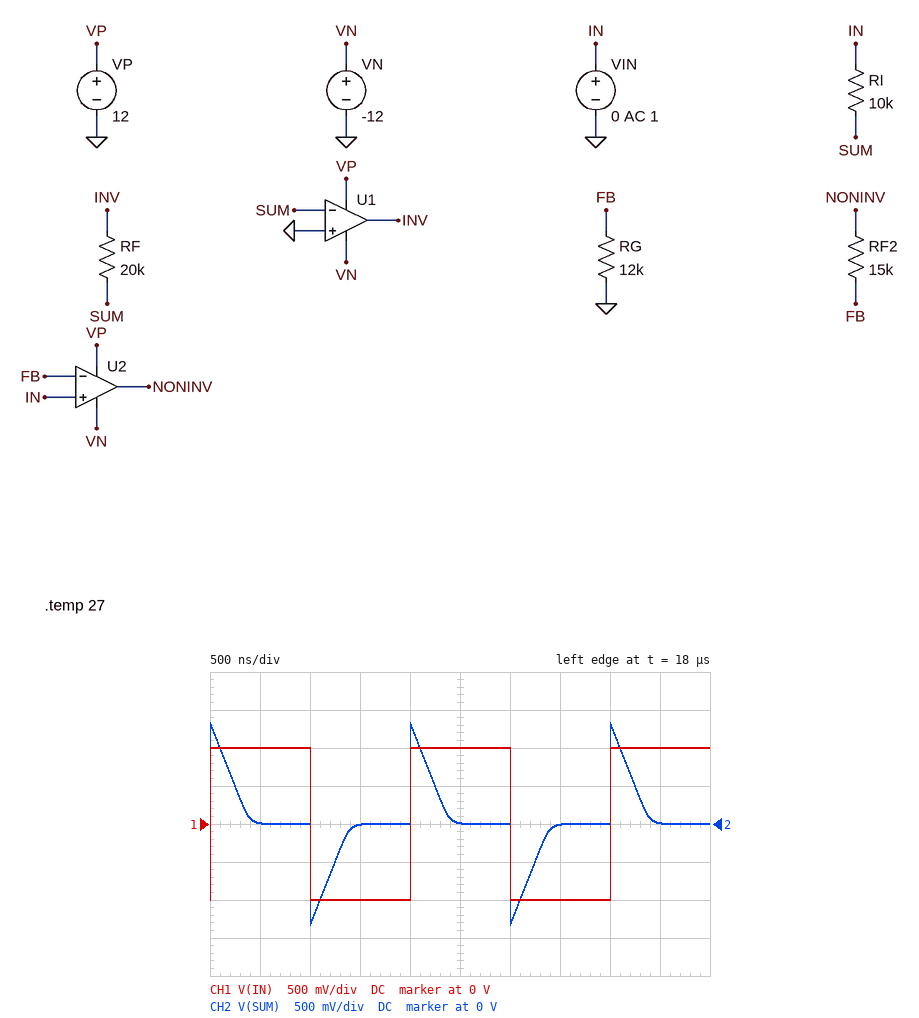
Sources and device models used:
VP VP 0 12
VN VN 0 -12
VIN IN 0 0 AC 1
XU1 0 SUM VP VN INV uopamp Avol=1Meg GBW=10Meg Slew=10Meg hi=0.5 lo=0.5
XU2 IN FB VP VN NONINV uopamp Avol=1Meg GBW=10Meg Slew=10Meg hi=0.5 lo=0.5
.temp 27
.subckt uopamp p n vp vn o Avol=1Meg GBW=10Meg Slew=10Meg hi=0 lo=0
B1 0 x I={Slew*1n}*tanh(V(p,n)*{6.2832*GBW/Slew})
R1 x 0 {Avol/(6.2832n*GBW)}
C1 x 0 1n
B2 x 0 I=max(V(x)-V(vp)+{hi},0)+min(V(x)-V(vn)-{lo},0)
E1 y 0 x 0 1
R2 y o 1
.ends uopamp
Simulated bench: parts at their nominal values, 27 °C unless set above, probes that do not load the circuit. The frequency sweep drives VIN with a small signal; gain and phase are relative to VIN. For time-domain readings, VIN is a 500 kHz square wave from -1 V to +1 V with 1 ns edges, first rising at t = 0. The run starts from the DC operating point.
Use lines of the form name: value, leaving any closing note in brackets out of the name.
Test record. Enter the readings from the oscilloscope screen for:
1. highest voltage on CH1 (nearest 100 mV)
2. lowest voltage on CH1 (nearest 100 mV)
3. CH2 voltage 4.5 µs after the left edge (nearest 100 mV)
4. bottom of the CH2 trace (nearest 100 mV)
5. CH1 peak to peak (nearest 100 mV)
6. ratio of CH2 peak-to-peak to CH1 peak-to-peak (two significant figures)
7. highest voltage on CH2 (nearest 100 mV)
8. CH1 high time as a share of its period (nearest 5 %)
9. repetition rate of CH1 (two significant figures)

highest voltage on CH1: 1.0 V
lowest voltage on CH1: -1.0 V
CH2 voltage 4.5 µs after the left edge: 0 V
bottom of the CH2 trace: -1.3 V
CH1 peak to peak: 2.0 V
ratio of CH2 peak-to-peak to CH1 peak-to-peak: 1.3
highest voltage on CH2: 1.3 V
CH1 high time as a share of its period: 50 %
repetition rate of CH1: 500 kHz
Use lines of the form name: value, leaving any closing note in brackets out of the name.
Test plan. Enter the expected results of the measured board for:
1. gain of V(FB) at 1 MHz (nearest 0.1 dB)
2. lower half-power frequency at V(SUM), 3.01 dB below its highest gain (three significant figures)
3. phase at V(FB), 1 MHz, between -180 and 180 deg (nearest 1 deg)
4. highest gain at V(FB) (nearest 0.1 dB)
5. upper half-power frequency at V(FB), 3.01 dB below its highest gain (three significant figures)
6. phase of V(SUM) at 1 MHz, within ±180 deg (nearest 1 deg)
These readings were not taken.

gain of V(FB) at 1 MHz: -0.2 dB
lower half-power frequency at V(SUM), 3.01 dB below its highest gain: 3.33 MHz
phase at V(FB), 1 MHz, between -180 and 180 deg: -13 deg
highest gain at V(FB): 0 dB
upper half-power frequency at V(FB), 3.01 dB below its highest gain: 4.44 MHz
phase of V(SUM) at 1 MHz, within ±180 deg: 73 deg
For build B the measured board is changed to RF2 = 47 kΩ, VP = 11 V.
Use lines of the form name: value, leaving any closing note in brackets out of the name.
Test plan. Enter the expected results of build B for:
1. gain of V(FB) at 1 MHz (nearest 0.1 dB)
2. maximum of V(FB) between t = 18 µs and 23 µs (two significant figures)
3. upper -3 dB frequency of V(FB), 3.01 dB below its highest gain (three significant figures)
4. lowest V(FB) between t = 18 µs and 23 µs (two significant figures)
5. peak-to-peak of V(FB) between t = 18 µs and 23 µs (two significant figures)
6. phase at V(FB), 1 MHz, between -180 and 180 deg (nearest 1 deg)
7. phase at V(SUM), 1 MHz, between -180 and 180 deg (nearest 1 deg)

gain of V(FB) at 1 MHz: -0.9 dB
maximum of V(FB) between t = 18 µs and 23 µs: 950 mV
upper -3 dB frequency of V(FB), 3.01 dB below its highest gain: 2.03 MHz
lowest V(FB) between t = 18 µs and 23 µs: -950 mV
peak-to-peak of V(FB) between t = 18 µs and 23 µs: 1.9 V
phase at V(FB), 1 MHz, between -180 and 180 deg: -26 deg
phase at V(SUM), 1 MHz, between -180 and 180 deg: 73 deg
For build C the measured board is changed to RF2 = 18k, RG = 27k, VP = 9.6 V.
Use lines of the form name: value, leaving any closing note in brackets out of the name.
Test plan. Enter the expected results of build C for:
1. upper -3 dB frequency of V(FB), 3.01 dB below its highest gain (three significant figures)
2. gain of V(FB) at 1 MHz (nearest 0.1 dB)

upper -3 dB frequency of V(FB), 3.01 dB below its highest gain: 6.00 MHz
gain of V(FB) at 1 MHz: -0.1 dB
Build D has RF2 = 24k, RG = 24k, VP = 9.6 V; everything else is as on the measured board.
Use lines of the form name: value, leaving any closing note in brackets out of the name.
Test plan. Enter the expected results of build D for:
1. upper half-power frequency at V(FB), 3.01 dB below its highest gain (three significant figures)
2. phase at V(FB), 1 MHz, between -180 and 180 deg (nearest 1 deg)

upper half-power frequency at V(FB), 3.01 dB below its highest gain: 5.00 MHz
phase at V(FB), 1 MHz, between -180 and 180 deg: -11 deg
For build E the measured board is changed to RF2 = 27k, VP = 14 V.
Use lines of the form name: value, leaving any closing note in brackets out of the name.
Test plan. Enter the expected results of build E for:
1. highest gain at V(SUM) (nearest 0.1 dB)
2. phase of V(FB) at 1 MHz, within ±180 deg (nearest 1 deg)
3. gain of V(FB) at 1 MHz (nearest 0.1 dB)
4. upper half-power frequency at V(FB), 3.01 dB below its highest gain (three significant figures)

highest gain at V(SUM): -3.5 dB
phase of V(FB) at 1 MHz, within ±180 deg: -18 deg
gain of V(FB) at 1 MHz: -0.4 dB
upper half-power frequency at V(FB), 3.01 dB below its highest gain: 3.08 MHz
